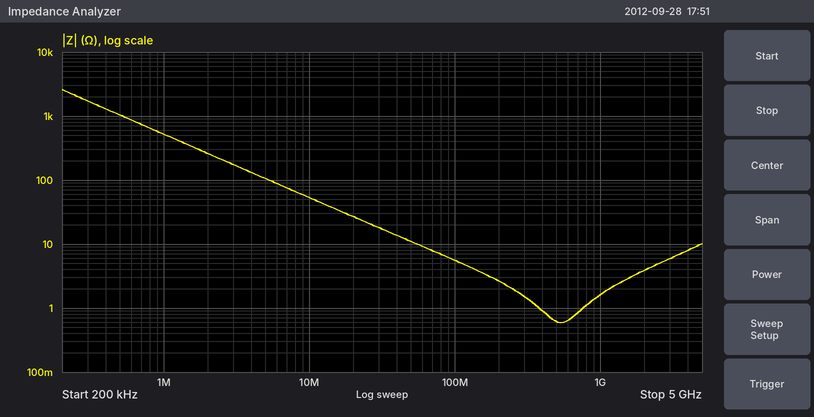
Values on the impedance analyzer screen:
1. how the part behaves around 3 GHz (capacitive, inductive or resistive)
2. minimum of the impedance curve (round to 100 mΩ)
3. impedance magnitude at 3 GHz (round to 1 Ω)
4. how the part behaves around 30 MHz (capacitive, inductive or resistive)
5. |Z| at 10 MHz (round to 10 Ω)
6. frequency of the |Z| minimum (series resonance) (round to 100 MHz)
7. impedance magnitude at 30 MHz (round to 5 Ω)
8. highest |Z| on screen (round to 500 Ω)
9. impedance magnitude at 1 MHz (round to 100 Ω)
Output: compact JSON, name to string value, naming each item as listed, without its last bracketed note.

{"how the part behaves around 3 GHz": "inductive", "minimum of the impedance curve": "600 mΩ", "impedance magnitude at 3 GHz": "6 Ω", "how the part behaves around 30 MHz": "capacitive", "|Z| at 10 MHz": "50 Ω", "frequency of the |Z| minimum (series resonance)": "500 MHz", "impedance magnitude at 30 MHz": "20 Ω", "highest |Z| on screen": "2.5 kΩ", "impedance magnitude at 1 MHz": "500 Ω"}
